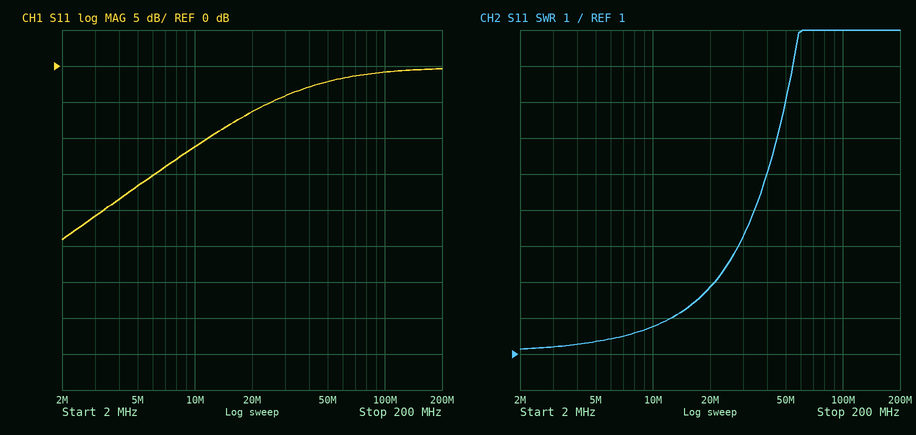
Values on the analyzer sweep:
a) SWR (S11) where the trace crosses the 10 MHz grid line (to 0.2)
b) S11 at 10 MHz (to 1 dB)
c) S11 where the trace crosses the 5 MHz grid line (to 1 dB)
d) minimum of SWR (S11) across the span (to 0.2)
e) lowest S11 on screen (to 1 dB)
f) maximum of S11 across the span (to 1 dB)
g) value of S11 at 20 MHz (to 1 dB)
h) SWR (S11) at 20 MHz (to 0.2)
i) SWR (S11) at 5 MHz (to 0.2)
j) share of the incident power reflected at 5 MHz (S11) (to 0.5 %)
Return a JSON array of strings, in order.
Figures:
["1.8", "-11 dB", "-17 dB", "1.2", "-24 dB", "0 dB", "-6 dB", "2.8", "1.4", "2.0 %"]
